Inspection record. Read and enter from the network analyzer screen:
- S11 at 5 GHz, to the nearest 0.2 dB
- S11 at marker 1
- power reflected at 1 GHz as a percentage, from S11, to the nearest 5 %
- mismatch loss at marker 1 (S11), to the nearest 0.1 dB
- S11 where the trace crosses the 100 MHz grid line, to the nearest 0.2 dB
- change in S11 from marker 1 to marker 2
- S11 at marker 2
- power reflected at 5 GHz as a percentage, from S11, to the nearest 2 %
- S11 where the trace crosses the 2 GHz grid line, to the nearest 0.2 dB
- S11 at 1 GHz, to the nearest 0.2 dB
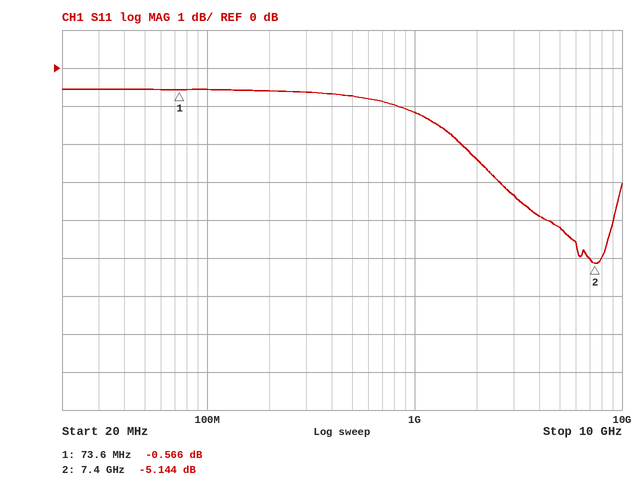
-4.2 dB
-0.566 dB
75 %
9.1 dB
-0.6 dB
-4.578 dB
-5.144 dB
38 %
-2.4 dB
-1.2 dB
